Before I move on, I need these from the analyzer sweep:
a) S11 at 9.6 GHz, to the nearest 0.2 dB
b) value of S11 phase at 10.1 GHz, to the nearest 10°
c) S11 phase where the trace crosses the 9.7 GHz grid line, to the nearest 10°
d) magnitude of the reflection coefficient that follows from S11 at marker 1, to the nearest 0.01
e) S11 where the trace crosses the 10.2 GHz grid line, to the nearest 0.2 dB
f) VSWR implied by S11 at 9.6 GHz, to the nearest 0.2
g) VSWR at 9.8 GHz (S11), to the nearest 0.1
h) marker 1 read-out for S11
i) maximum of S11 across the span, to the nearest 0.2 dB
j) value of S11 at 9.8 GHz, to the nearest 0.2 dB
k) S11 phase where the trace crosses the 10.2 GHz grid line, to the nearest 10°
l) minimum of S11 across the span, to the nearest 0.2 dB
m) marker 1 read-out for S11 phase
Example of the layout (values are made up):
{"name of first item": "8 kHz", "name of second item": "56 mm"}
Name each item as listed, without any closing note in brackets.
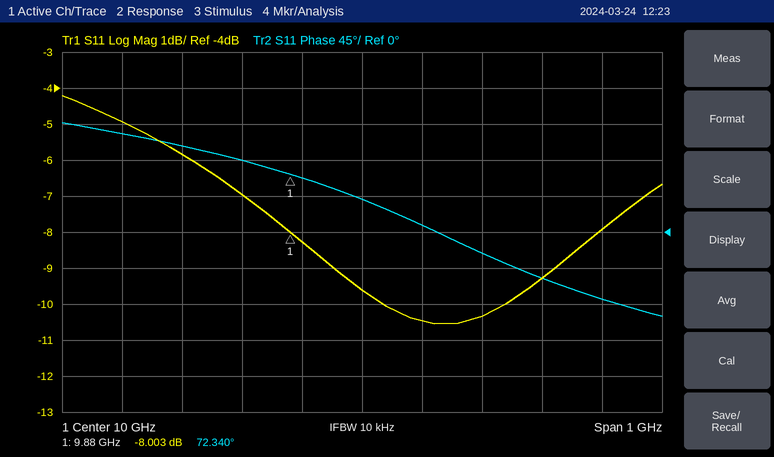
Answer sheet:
{"S11 at 9.6 GHz, to the nearest 0.2 dB": "-5.0 dB", "value of S11 phase at 10.1 GHz, to the nearest 10°": "10°", "S11 phase where the trace crosses the 9.7 GHz grid line, to the nearest 10°": "110°", "magnitude of the reflection coefficient that follows from S11 at marker 1, to the nearest 0.01": "0.40", "S11 where the trace crosses the 10.2 GHz grid line, to the nearest 0.2 dB": "-10.4 dB", "VSWR implied by S11 at 9.6 GHz, to the nearest 0.2": "3.6", "VSWR at 9.8 GHz (S11), to the nearest 0.1": "2.6", "marker 1 read-out for S11": "-8.003 dB", "maximum of S11 across the span, to the nearest 0.2 dB": "-4.2 dB", "value of S11 at 9.8 GHz, to the nearest 0.2 dB": "-7.0 dB", "S11 phase where the trace crosses the 10.2 GHz grid line, to the nearest 10°": "-30°", "minimum of S11 across the span, to the nearest 0.2 dB": "-10.6 dB", "marker 1 read-out for S11 phase": "72.340°"}
